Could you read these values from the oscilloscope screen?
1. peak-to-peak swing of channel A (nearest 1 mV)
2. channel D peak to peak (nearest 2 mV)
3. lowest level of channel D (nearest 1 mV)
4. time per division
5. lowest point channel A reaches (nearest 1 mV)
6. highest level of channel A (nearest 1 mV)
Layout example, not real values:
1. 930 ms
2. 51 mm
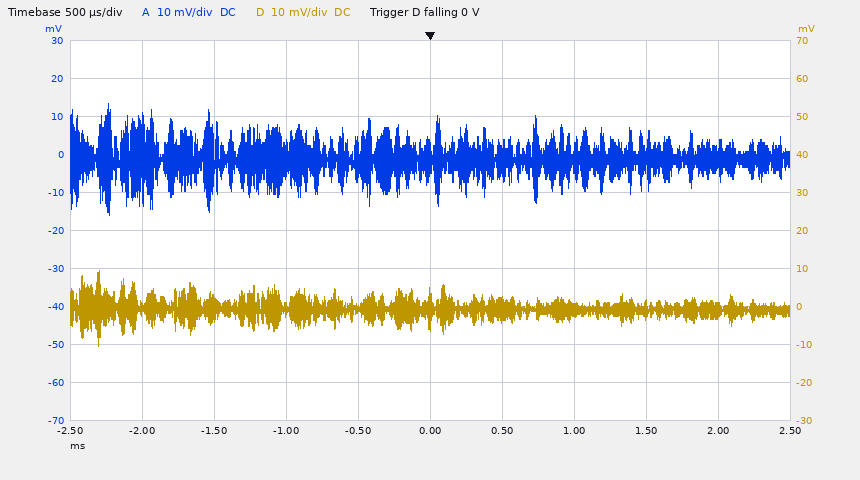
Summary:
1. 29 mV
2. 20 mV
3. -10 mV
4. 500 µs
5. -16 mV
6. 13 mV
